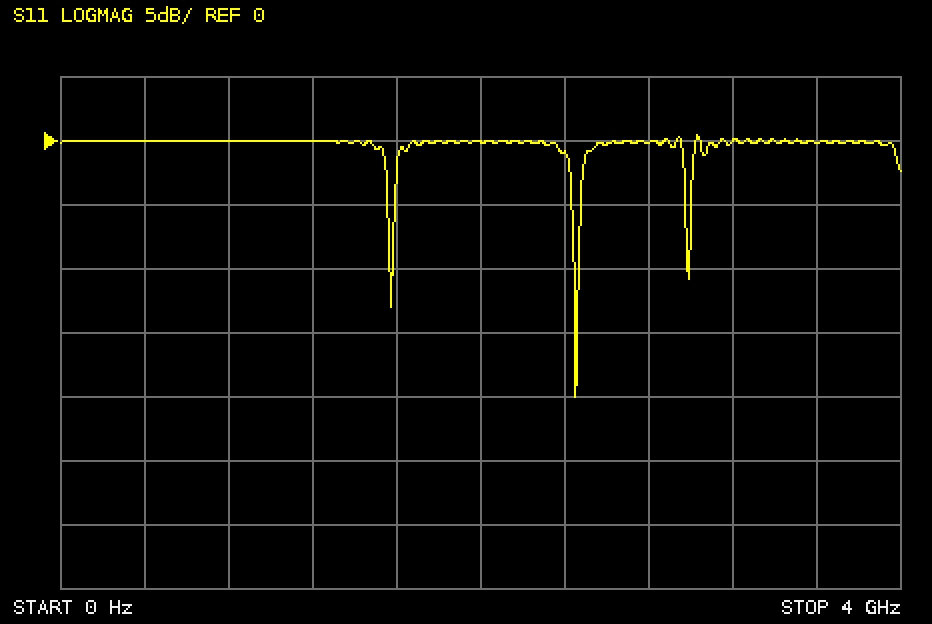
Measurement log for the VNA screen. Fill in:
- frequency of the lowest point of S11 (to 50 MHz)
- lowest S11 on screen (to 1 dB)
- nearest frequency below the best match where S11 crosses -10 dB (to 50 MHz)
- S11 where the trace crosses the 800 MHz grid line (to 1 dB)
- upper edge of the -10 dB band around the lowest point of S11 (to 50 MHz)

2.45 GHz
-20 dB
2.45 GHz
0 dB
2.45 GHz
